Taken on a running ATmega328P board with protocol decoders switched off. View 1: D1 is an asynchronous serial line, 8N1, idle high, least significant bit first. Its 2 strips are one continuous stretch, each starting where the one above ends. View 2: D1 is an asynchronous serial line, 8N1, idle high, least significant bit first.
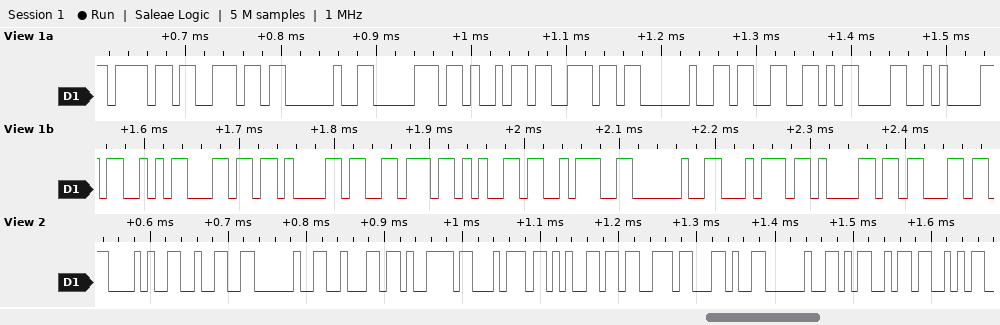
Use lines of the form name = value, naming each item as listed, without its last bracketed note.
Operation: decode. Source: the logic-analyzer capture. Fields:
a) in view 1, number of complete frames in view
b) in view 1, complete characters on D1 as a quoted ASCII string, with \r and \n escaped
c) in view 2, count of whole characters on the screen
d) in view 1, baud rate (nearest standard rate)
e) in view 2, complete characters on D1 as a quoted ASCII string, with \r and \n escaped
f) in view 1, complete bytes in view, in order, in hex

in view 1, number of complete frames in view = 20
in view 1, complete characters on D1 as a quoted ASCII string, with \r and \n escaped = "on pin 3\r\nSlave: tac"
in view 2, count of whole characters on the screen = 12
in view 1, baud rate = 115200 baud
in view 2, complete characters on D1 as a quoted ASCII string, with \r and \n escaped = "(2 bytes, MS"
in view 1, complete bytes in view, in order, in hex = 6F 6E 20 70 69 6E 20 33 0D 0A 53 6C 61 76 65 3A 20 74 61 63
